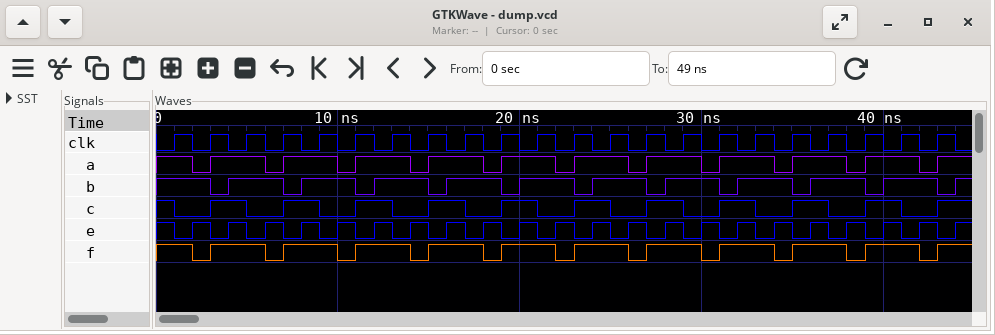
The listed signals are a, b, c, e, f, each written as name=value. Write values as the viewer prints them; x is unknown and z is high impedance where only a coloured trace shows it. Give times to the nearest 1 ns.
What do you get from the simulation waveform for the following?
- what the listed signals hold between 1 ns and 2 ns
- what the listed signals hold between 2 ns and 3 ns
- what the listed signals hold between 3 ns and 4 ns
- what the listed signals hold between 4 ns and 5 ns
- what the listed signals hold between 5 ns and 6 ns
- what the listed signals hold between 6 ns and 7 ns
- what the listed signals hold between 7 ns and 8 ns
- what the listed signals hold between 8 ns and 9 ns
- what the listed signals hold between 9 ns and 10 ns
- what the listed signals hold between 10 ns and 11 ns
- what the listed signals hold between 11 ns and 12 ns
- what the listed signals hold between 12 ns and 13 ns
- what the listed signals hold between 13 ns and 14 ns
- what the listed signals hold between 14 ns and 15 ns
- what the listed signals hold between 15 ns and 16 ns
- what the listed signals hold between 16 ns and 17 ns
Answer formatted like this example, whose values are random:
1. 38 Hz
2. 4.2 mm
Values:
1. a=1, b=1, c=0, e=0, f=1
2. a=0, b=1, c=0, e=1, f=0
3. a=1, b=0, c=1, e=0, f=1
4. a=1, b=1, c=1, e=1, f=1
5. a=1, b=1, c=0, e=0, f=1
6. a=0, b=1, c=0, e=1, f=0
7. a=1, b=0, c=1, e=0, f=1
8. a=1, b=1, c=1, e=1, f=1
9. a=1, b=1, c=0, e=0, f=1
10. a=0, b=1, c=0, e=1, f=0
11. a=1, b=0, c=1, e=0, f=1
12. a=1, b=1, c=1, e=1, f=1
13. a=1, b=1, c=0, e=0, f=1
14. a=0, b=1, c=0, e=1, f=0
15. a=1, b=0, c=1, e=0, f=1
16. a=1, b=1, c=1, e=1, f=1
